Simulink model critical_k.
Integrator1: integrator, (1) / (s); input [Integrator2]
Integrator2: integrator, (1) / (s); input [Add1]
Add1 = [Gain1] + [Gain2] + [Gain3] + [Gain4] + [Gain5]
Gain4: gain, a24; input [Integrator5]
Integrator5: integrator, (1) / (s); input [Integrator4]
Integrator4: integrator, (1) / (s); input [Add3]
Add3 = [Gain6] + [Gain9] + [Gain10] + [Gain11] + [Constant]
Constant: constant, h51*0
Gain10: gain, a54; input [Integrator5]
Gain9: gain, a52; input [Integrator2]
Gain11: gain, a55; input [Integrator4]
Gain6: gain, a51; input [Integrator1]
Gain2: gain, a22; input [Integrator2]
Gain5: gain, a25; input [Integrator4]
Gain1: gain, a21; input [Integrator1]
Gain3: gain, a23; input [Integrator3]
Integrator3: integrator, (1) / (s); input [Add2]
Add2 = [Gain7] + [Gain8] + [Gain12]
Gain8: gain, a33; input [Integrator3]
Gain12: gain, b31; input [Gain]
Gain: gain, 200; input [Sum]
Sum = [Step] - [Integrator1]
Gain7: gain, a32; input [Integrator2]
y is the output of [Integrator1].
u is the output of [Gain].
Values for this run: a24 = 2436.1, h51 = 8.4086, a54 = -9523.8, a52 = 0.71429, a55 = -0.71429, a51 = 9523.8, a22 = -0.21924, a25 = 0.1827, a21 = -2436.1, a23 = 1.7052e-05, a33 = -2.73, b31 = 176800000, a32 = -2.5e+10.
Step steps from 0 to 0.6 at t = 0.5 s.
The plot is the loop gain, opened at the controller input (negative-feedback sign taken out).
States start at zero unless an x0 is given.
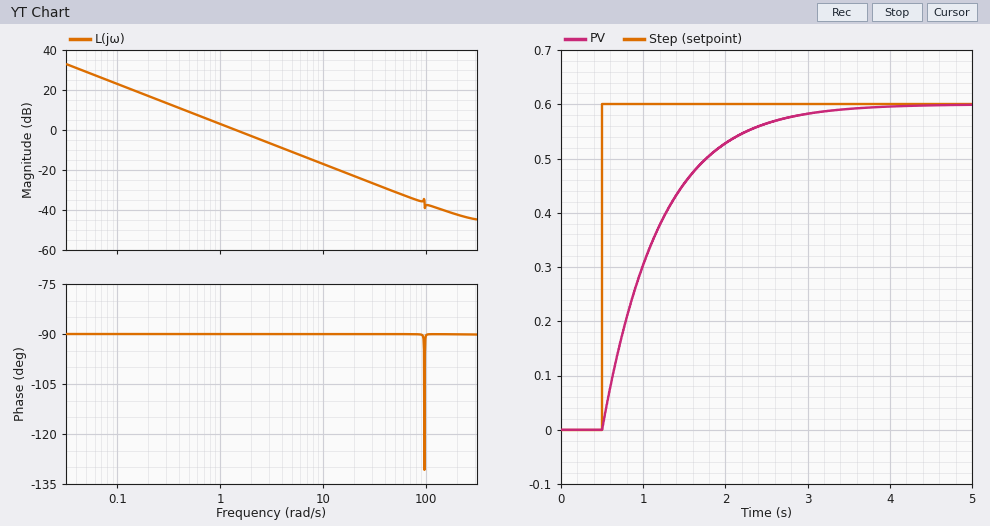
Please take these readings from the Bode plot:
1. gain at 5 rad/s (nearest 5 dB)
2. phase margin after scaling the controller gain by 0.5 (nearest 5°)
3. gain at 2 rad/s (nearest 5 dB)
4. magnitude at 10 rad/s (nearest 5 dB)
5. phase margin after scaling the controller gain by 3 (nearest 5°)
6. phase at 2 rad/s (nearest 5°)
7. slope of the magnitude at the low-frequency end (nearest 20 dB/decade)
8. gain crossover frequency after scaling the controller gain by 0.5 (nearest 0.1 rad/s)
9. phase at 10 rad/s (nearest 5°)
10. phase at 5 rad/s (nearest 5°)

-10 dB
90°
-5 dB
-15 dB
90°
-90°
-20 dB/decade
0.7 rad/s
-90°
-90°
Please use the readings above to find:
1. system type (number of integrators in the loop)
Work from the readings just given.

1
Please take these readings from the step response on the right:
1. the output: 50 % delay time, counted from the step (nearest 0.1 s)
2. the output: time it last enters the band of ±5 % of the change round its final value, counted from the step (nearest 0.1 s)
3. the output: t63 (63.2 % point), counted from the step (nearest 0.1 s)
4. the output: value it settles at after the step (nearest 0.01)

0.5 s
2.1 s
0.7 s
0.60
